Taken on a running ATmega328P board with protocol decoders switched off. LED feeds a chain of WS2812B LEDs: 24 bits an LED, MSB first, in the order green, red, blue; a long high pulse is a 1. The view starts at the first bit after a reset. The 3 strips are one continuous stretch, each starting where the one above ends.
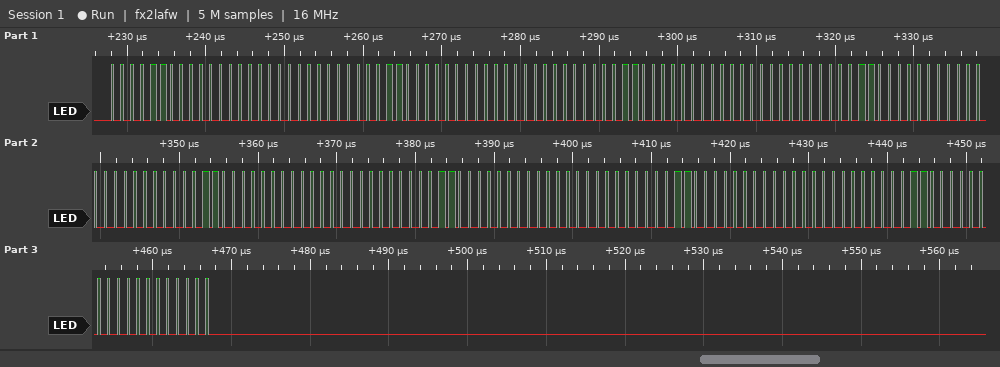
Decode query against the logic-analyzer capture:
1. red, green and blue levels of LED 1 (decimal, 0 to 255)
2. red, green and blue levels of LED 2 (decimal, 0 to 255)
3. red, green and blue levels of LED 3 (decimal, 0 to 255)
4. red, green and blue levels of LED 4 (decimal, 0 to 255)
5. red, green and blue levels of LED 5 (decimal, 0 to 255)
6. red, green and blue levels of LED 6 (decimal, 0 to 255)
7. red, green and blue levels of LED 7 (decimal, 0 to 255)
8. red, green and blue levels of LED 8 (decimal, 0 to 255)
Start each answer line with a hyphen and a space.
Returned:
- 0, 12, 0
- 0, 12, 0
- 0, 12, 0
- 0, 12, 0
- 0, 12, 0
- 0, 12, 0
- 0, 12, 0
- 0, 12, 0
